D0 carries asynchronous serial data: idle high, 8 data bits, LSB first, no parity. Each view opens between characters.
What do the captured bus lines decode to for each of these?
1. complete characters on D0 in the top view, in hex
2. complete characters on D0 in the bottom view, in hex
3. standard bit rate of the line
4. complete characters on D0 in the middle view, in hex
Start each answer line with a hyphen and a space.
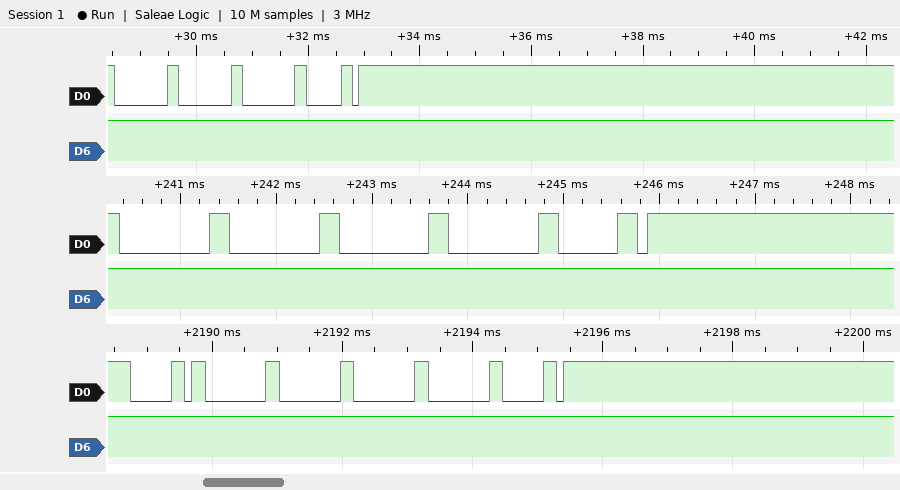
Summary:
- 00, 00, 00, 60
- 60, 00, 00, 00, 00, 60
- 9600 baud
- 00, 00, 00, 00, 60
